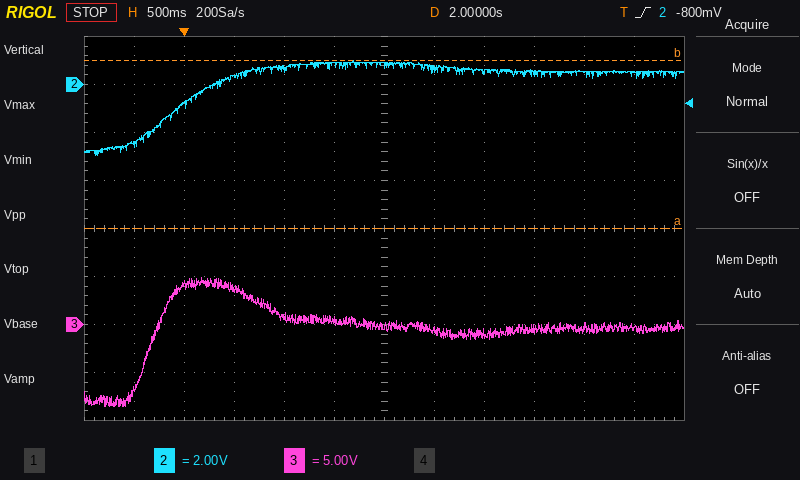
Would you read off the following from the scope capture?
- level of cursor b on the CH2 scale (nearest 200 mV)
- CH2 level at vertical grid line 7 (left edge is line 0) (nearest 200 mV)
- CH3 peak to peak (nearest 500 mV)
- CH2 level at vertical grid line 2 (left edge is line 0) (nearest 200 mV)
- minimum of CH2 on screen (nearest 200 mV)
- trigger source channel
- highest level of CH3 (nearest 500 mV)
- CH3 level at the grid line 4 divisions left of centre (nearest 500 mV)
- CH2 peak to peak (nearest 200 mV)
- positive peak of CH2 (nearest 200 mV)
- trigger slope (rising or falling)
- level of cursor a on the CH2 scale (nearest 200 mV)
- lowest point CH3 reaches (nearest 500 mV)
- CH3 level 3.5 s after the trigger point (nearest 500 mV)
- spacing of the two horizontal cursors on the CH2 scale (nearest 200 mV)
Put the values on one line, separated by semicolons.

1.0 V; 600 mV; 13.5 V; -800 mV; -3.0 V; CH2; 5.0 V; 4.0 V; 4.0 V; 1.0 V; rising; -6.0 V; -8.5 V; -500 mV; 7.0 V
